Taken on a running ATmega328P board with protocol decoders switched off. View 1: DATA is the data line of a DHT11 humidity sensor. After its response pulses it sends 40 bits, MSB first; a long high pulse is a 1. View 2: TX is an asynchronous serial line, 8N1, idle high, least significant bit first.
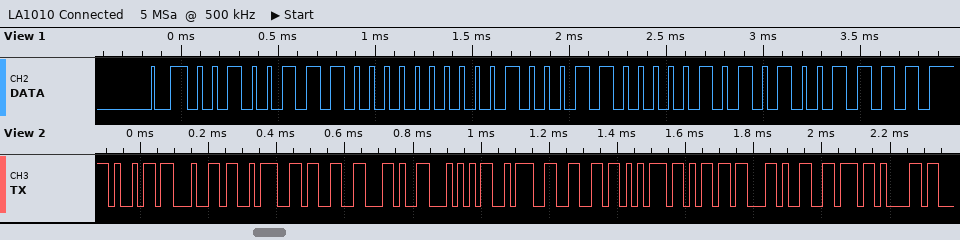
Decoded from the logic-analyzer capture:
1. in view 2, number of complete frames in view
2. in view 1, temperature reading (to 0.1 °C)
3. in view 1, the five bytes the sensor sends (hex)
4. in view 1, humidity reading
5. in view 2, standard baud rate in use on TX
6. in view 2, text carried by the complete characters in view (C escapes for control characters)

13
35.5 °C
27 00 23 05 4F
39 %
57600 baud
"id:3,T:fum,va"
